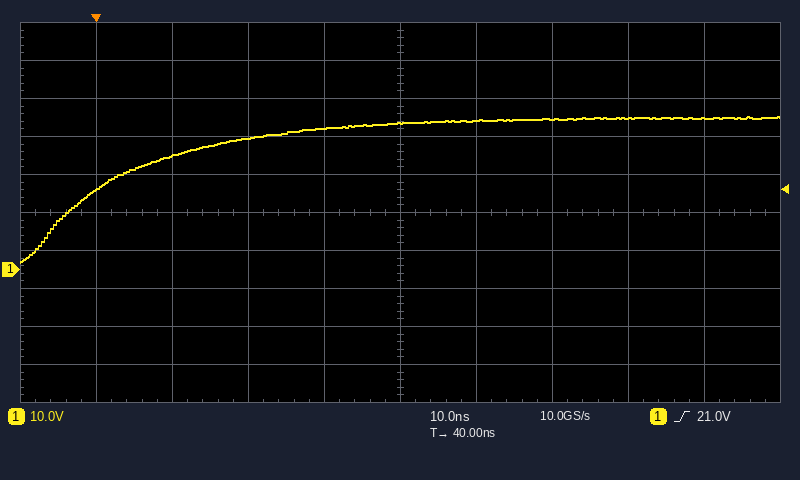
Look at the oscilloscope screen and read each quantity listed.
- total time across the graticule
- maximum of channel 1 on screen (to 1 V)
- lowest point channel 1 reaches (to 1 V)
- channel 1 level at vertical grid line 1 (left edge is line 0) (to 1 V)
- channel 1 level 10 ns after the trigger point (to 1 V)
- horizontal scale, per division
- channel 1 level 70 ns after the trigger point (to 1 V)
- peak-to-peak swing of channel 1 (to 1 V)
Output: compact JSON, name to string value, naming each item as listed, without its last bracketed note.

{"total time across the graticule": "100 ns", "maximum of channel 1 on screen": "40 V", "lowest point channel 1 reaches": "2 V", "channel 1 level at vertical grid line 1 (left edge is line 0)": "21 V", "channel 1 level 10 ns after the trigger point": "30 V", "horizontal scale, per division": "10 ns", "channel 1 level 70 ns after the trigger point": "40 V", "peak-to-peak swing of channel 1": "38 V"}
